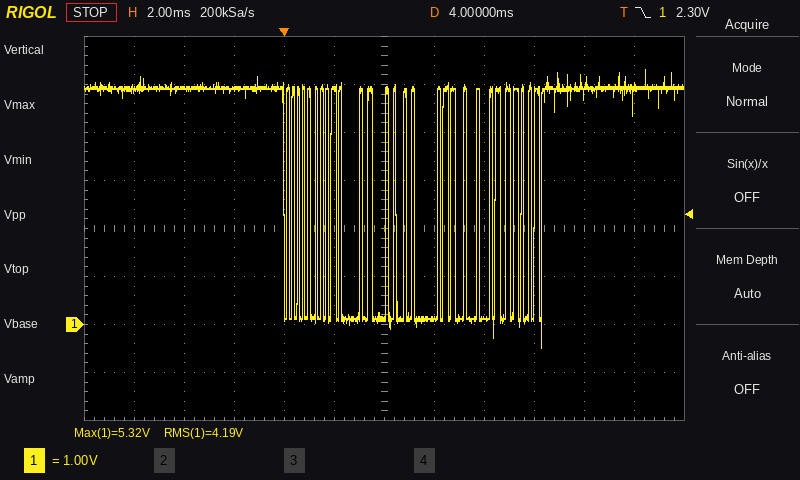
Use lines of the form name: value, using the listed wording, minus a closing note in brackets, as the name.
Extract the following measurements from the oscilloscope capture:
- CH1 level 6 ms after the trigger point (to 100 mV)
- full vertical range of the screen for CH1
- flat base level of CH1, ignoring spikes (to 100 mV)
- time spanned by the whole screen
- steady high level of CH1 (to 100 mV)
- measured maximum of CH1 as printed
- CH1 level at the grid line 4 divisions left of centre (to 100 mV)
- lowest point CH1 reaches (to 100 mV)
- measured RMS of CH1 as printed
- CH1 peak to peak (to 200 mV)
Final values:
CH1 level 6 ms after the trigger point: 100 mV
full vertical range of the screen for CH1: 8 V
flat base level of CH1, ignoring spikes: 100 mV
time spanned by the whole screen: 24 ms
steady high level of CH1: 4.9 V
measured maximum of CH1 as printed: 5.32 V
CH1 level at the grid line 4 divisions left of centre: 4.9 V
lowest point CH1 reaches: -500 mV
measured RMS of CH1 as printed: 4.19 V
CH1 peak to peak: 5.8 V
